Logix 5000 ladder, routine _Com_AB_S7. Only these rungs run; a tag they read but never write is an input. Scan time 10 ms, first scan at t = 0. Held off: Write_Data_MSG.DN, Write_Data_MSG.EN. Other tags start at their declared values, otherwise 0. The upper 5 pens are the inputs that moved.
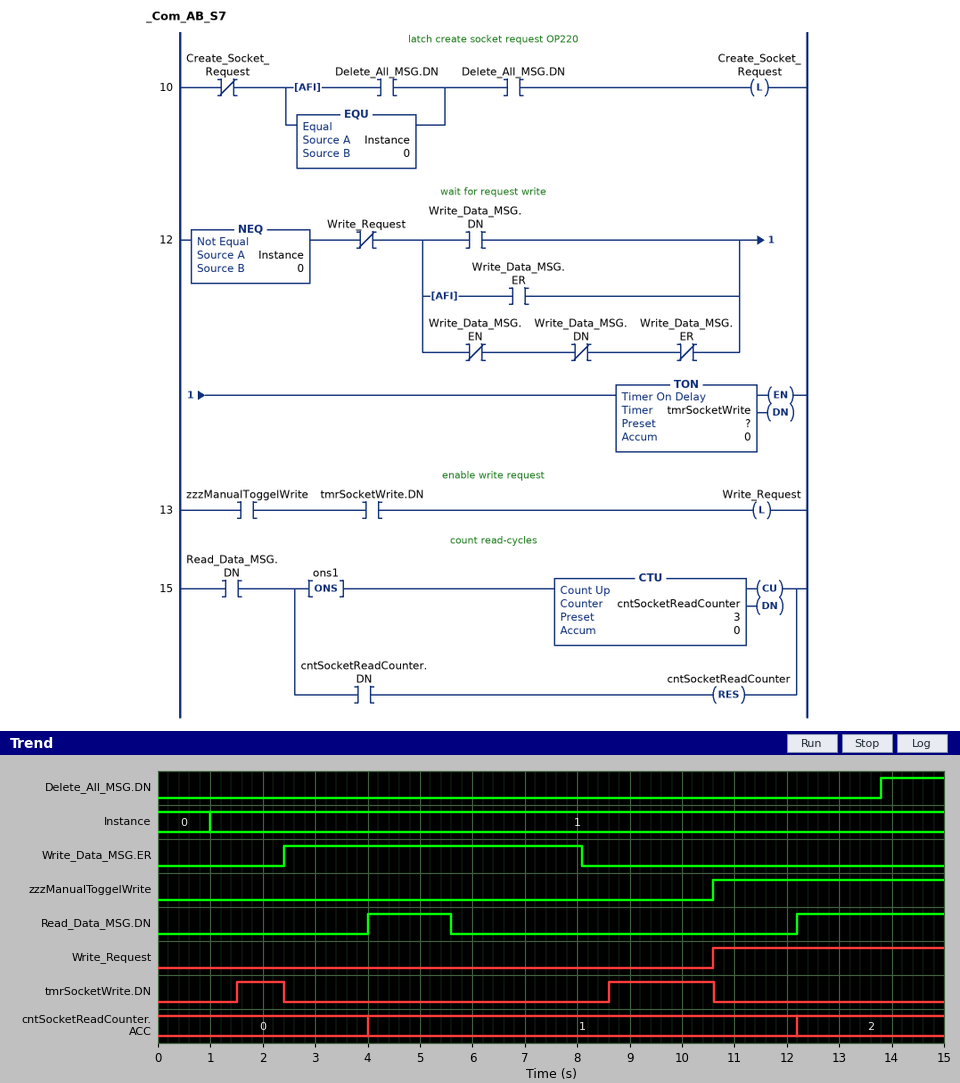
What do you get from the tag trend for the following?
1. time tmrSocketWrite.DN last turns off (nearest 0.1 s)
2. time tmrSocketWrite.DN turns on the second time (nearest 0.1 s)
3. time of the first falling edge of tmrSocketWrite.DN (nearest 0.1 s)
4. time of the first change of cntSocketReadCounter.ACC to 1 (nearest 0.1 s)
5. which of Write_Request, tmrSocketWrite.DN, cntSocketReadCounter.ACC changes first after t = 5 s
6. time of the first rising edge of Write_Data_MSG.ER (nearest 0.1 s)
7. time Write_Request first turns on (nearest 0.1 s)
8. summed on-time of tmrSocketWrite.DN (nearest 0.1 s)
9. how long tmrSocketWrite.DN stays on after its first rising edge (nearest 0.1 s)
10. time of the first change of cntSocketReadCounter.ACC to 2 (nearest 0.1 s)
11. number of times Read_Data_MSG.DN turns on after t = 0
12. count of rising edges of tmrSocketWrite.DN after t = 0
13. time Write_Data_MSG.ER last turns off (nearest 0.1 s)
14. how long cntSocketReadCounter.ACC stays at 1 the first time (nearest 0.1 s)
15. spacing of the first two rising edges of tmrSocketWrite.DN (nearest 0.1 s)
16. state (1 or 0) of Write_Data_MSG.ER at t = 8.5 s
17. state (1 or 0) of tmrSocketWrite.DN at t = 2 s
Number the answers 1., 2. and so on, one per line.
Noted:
1. 10.6 s
2. 8.6 s
3. 2.4 s
4. 4.0 s
5. tmrSocketWrite.DN
6. 2.4 s
7. 10.6 s
8. 2.9 s
9. 0.9 s
10. 12.2 s
11. 2
12. 2
13. 8.1 s
14. 8.2 s
15. 7.1 s
16. 0
17. 1
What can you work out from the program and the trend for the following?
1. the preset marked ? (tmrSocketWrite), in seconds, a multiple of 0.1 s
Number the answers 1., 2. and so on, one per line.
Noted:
1. 0.5 s
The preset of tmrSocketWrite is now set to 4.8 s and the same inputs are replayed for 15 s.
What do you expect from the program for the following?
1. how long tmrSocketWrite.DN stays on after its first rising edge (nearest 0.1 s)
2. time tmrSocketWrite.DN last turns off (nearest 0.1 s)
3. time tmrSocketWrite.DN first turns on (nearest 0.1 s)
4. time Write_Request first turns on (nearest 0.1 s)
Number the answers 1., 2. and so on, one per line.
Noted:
1. 0.0 s
2. 12.9 s
3. 12.9 s
4. 12.9 s
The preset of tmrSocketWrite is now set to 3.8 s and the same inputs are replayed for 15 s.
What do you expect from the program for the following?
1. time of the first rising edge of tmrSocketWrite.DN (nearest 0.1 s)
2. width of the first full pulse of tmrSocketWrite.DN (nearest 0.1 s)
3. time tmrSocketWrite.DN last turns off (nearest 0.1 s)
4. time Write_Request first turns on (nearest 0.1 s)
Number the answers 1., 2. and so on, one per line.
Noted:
1. 11.9 s
2. 0.0 s
3. 11.9 s
4. 11.9 s
